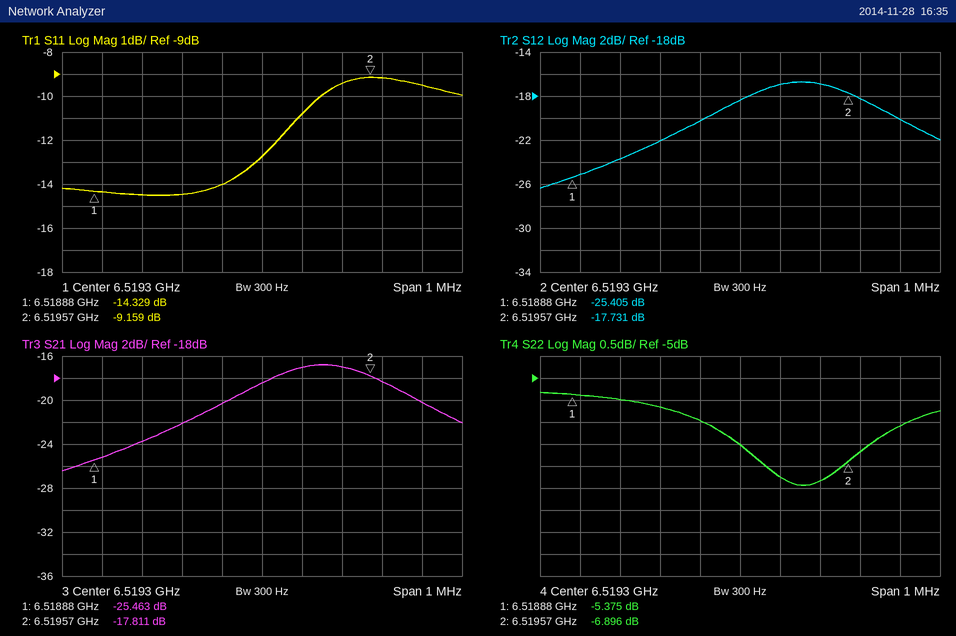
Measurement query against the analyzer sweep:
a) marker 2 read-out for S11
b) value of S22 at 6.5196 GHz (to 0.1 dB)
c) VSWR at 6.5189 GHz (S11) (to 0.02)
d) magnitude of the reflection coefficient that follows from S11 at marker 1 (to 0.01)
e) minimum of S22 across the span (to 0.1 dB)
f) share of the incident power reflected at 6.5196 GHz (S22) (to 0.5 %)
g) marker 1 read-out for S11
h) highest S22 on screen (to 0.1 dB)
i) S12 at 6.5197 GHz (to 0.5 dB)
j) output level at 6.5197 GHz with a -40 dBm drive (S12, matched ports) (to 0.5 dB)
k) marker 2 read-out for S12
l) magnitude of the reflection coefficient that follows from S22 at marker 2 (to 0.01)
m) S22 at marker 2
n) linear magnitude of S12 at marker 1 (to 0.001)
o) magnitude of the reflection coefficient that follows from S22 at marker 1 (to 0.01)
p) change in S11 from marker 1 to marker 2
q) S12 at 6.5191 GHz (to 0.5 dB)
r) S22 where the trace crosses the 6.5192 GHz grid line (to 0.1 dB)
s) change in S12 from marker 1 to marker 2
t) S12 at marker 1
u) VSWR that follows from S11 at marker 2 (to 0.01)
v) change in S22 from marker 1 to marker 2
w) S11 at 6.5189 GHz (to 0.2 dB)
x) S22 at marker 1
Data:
-9.159 dB
-6.7 dB
1.48
0.19
-7.4 dB
21.5 %
-14.329 dB
-5.3 dB
-20.0 dB
-60.0 dBm
-17.731 dB
0.45
-6.896 dB
0.054
0.54
5.170 dB
-22.0 dB
-6.0 dB
7.674 dB
-25.405 dB
2.07
-1.521 dB
-14.4 dB
-5.375 dB
